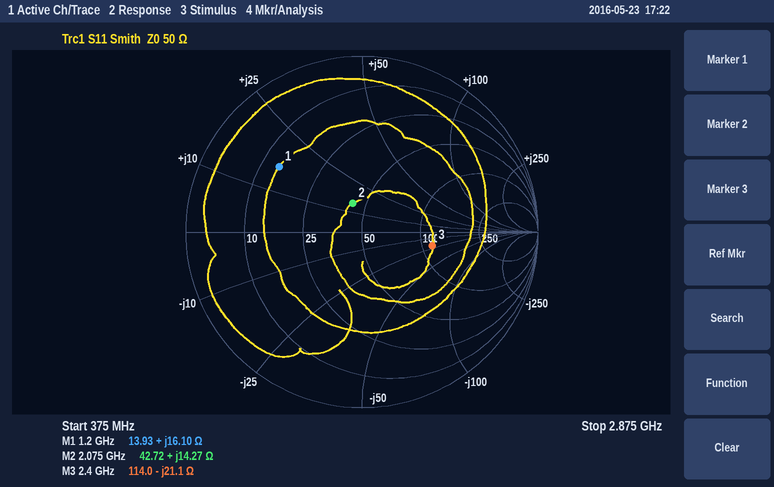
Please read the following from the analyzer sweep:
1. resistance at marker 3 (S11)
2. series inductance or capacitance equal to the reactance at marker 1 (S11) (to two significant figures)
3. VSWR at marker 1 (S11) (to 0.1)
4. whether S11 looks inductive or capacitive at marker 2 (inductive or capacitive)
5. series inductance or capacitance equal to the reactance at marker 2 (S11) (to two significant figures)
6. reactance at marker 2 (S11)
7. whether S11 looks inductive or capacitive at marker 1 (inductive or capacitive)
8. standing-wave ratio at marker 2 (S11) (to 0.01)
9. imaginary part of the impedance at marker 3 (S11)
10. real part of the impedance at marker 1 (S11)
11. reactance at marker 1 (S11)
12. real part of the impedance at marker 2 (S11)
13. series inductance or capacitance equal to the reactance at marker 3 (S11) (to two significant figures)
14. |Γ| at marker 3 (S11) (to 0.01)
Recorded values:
114.0 Ω
2.1 nH
4.0
inductive
1.1 nH
+14.27 Ω
inductive
1.41
-21.1 Ω
13.93 Ω
+16.10 Ω
42.72 Ω
3.1 pF
0.41
